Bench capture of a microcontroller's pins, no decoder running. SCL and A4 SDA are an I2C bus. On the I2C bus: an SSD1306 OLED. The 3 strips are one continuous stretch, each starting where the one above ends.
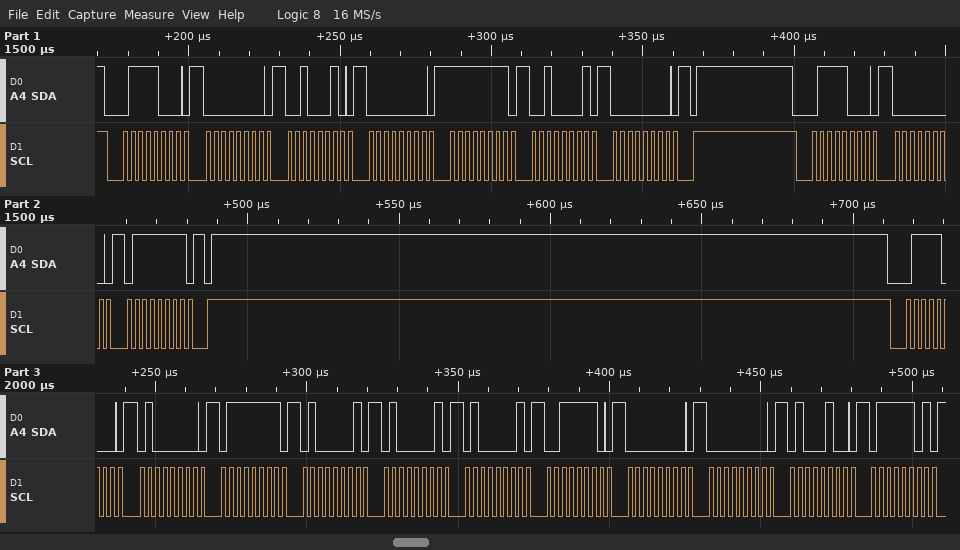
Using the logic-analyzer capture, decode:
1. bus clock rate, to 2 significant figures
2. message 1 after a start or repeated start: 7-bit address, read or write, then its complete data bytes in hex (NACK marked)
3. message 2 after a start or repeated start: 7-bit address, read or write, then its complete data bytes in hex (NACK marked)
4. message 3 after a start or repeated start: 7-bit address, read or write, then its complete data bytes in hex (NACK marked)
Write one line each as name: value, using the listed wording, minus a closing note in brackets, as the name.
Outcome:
bus clock rate, to 2 significant figures: 400 kHz
message 1 after a start or repeated start: 7-bit address, read or write, then its complete data bytes in hex: 0x3C write: 00 22 00 FF 21 00
message 2 after a start or repeated start: 7-bit address, read or write, then its complete data bytes in hex: 0x3C write: 00 7F
message 3 after a start or repeated start: 7-bit address, read or write, then its complete data bytes in hex: 0x3C write: 40 7F 41 41 41 3E 00 00 44 7D
